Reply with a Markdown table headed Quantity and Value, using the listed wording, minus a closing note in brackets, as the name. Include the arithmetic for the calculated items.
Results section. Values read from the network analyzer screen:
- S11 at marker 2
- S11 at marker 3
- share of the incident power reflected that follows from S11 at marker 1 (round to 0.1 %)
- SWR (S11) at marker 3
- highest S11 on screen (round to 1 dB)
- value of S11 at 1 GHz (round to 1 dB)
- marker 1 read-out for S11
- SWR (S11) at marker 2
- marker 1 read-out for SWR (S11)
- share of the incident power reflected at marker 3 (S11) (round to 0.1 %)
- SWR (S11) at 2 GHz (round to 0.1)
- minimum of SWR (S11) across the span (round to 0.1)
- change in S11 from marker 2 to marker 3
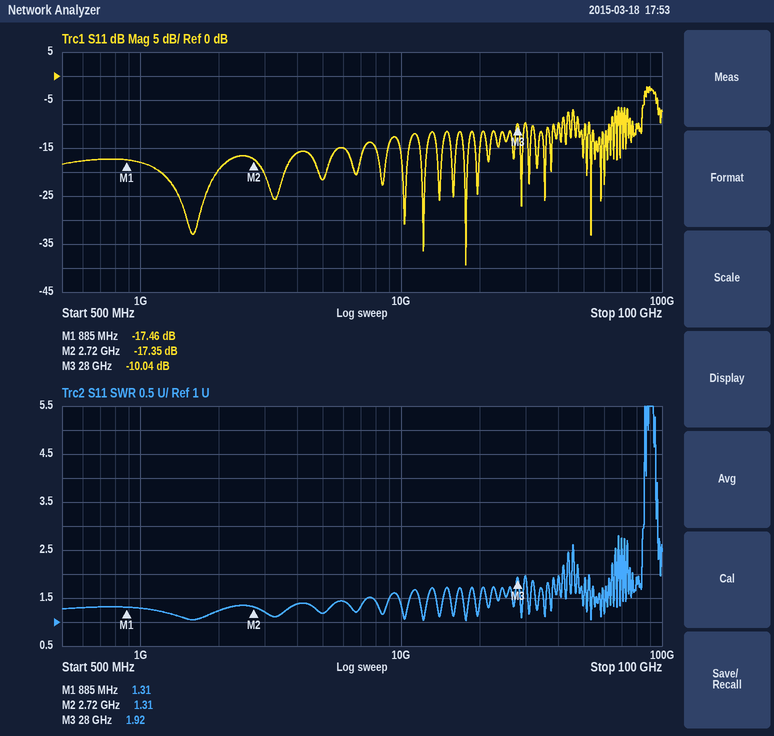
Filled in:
| Quantity | Value |
|---|---|
| S11 at marker 2 | -17.35 dB |
| S11 at marker 3 | -10.04 dB |
| share of the incident power reflected that follows from S11 at marker 1 | 10^(-17.46/10) ≈ 1.8 % |
| SWR (S11) at marker 3 | 1.92 |
| highest S11 on screen | -2 dB |
| value of S11 at 1 GHz | -18 dB |
| marker 1 read-out for S11 | -17.46 dB |
| SWR (S11) at marker 2 | 1.31 |
| marker 1 read-out for SWR | 1.31 |
| share of the incident power reflected at marker 3 (S11) | 10^(-10.04/10) ≈ 9.9 % |
| SWR (S11) at 2 GHz | 1.2 |
| minimum of SWR (S11) across the span | 1.0 |
| change in S11 from marker 2 to marker 3 | -10.04 − (-17.35) = 7.31 dB |
